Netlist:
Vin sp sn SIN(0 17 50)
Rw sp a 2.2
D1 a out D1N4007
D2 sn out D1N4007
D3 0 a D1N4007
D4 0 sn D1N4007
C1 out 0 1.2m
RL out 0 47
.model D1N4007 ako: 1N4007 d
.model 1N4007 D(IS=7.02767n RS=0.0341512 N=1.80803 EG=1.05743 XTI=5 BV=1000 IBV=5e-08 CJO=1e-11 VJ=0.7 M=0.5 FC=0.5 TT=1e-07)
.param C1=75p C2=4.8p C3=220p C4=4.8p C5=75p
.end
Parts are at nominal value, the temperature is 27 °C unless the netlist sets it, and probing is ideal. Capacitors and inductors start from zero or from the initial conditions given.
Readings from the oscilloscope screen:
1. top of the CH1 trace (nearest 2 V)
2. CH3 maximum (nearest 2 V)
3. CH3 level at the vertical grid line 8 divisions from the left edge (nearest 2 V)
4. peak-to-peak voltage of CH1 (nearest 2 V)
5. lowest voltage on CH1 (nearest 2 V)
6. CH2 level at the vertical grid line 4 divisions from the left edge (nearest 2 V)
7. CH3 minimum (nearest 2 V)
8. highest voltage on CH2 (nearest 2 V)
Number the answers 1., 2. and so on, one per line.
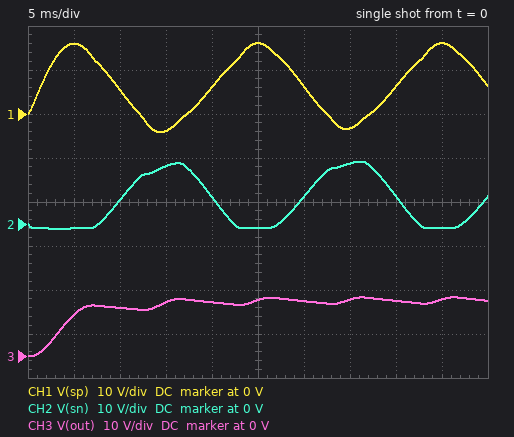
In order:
1. 16 V
2. 14 V
3. 12 V
4. 20 V
5. -4 V
6. 6 V
7. 0 V
8. 14 V
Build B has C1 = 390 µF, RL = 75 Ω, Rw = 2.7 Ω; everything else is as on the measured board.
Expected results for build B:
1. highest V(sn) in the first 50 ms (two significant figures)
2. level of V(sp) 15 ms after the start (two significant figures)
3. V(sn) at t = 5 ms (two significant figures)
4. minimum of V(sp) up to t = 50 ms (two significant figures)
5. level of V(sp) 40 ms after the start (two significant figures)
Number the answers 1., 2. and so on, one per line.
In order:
1. 15 V
2. -2.4 V
3. -890 mV
4. -2.9 V
5. 6.2 V
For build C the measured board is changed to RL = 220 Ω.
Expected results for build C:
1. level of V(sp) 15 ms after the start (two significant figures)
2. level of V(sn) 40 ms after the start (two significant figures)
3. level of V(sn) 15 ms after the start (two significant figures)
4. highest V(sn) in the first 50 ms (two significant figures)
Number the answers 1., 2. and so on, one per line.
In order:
1. -3.1 V
2. 7.1 V
3. 14 V
4. 15 V
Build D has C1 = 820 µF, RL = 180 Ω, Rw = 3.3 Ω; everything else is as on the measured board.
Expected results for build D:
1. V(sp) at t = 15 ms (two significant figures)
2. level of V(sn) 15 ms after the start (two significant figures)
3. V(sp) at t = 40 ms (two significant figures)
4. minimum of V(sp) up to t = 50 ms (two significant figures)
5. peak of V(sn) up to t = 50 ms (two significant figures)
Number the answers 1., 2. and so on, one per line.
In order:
1. -3.3 V
2. 14 V
3. 6.9 V
4. -3.6 V
5. 15 V
